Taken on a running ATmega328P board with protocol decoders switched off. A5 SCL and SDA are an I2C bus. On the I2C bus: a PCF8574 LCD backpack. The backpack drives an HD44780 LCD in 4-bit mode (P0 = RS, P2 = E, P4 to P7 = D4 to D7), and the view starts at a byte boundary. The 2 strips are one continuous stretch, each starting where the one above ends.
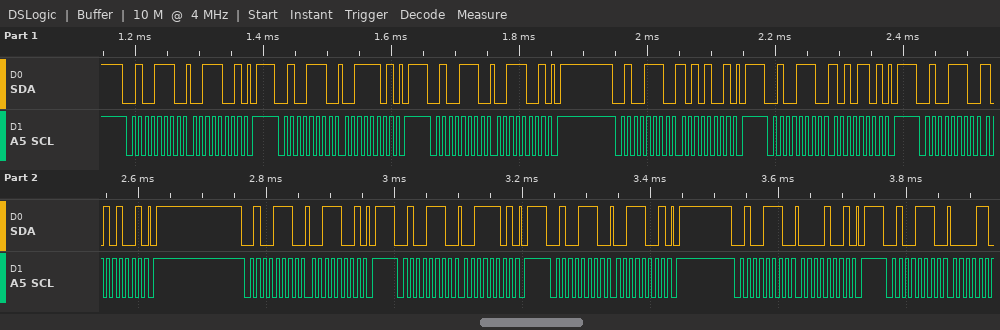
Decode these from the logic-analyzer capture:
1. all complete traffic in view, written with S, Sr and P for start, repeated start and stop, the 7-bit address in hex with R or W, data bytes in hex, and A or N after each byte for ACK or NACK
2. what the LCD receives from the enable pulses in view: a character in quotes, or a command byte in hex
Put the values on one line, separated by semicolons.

S 27W A 39 A P S 27W A 3D A P S 27W A 39 A P S 27W A A9 A P S 27W A AD A P S 27W A A9 A P S 27W A 39 A P S 27W A 3D A P S 27W A 39 A P S 27W A 09 A P S 27W A; ':'
